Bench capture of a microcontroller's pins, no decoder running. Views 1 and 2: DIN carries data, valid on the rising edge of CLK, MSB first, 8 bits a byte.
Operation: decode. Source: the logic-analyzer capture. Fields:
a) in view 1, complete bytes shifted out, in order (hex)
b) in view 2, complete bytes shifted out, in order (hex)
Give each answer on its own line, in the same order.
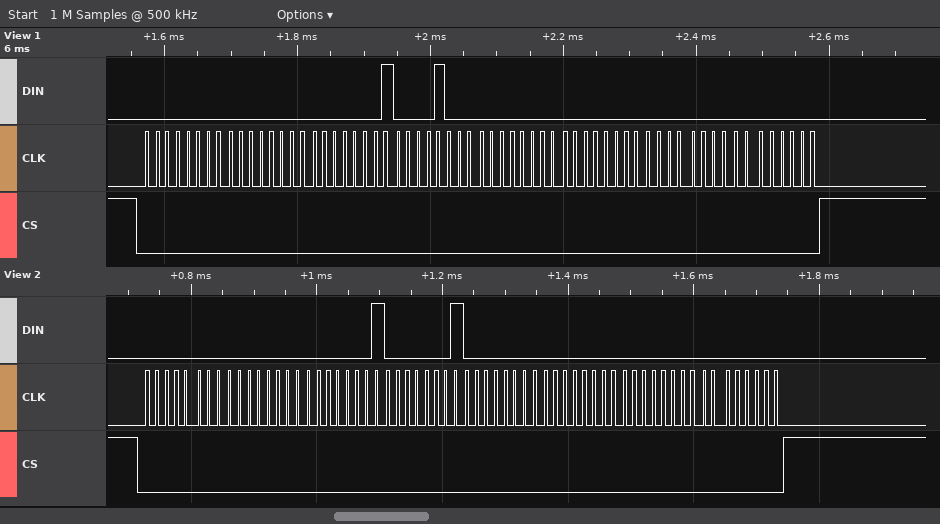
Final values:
0x00 0x00 0x01 0x08 0x00 0x00 0x00 0x00
00 00 01 01 00 00 00 00
